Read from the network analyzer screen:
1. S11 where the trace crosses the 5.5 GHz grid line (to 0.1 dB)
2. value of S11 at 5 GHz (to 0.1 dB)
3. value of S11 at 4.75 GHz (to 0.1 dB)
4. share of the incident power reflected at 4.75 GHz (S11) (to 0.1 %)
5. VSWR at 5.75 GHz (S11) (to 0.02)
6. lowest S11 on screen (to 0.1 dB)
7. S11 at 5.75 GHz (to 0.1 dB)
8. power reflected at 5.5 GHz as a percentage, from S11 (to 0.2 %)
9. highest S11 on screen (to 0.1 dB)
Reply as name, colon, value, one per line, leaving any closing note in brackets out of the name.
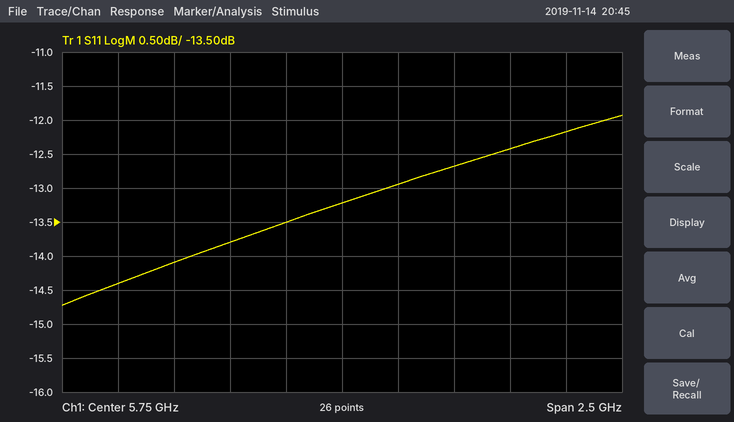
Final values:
S11 where the trace crosses the 5.5 GHz grid line: -13.5 dB
value of S11 at 5 GHz: -14.1 dB
value of S11 at 4.75 GHz: -14.4 dB
share of the incident power reflected at 4.75 GHz (S11): 3.6 %
VSWR at 5.75 GHz (S11): 1.56
lowest S11 on screen: -14.7 dB
S11 at 5.75 GHz: -13.2 dB
power reflected at 5.5 GHz as a percentage, from S11: 4.4 %
highest S11 on screen: -11.9 dB
